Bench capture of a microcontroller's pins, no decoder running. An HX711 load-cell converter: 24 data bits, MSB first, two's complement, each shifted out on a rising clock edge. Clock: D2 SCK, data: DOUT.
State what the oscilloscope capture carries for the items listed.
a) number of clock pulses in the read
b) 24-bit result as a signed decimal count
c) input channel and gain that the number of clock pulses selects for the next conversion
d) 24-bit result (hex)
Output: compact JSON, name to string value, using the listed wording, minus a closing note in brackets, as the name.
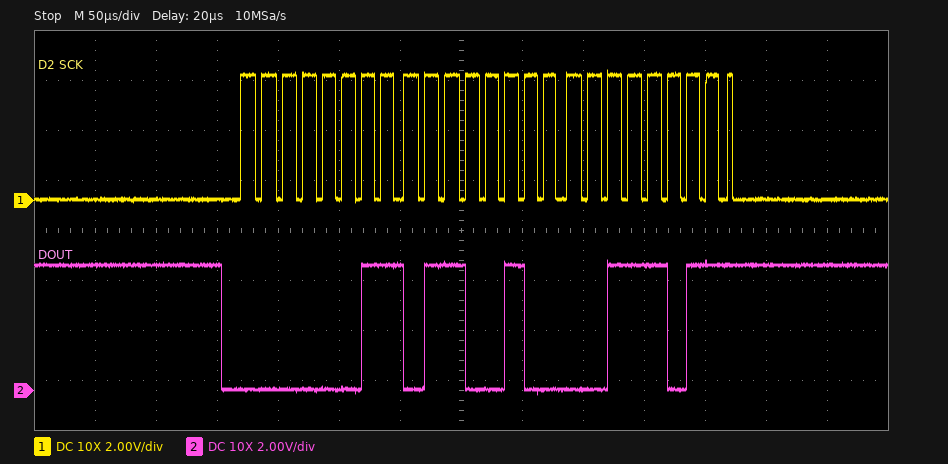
{"number of clock pulses in the read": "25", "24-bit result as a signed decimal count": "222267", "input channel and gain that the number of clock pulses selects for the next conversion": "channel A, gain 128", "24-bit result": "0x03643B"}
